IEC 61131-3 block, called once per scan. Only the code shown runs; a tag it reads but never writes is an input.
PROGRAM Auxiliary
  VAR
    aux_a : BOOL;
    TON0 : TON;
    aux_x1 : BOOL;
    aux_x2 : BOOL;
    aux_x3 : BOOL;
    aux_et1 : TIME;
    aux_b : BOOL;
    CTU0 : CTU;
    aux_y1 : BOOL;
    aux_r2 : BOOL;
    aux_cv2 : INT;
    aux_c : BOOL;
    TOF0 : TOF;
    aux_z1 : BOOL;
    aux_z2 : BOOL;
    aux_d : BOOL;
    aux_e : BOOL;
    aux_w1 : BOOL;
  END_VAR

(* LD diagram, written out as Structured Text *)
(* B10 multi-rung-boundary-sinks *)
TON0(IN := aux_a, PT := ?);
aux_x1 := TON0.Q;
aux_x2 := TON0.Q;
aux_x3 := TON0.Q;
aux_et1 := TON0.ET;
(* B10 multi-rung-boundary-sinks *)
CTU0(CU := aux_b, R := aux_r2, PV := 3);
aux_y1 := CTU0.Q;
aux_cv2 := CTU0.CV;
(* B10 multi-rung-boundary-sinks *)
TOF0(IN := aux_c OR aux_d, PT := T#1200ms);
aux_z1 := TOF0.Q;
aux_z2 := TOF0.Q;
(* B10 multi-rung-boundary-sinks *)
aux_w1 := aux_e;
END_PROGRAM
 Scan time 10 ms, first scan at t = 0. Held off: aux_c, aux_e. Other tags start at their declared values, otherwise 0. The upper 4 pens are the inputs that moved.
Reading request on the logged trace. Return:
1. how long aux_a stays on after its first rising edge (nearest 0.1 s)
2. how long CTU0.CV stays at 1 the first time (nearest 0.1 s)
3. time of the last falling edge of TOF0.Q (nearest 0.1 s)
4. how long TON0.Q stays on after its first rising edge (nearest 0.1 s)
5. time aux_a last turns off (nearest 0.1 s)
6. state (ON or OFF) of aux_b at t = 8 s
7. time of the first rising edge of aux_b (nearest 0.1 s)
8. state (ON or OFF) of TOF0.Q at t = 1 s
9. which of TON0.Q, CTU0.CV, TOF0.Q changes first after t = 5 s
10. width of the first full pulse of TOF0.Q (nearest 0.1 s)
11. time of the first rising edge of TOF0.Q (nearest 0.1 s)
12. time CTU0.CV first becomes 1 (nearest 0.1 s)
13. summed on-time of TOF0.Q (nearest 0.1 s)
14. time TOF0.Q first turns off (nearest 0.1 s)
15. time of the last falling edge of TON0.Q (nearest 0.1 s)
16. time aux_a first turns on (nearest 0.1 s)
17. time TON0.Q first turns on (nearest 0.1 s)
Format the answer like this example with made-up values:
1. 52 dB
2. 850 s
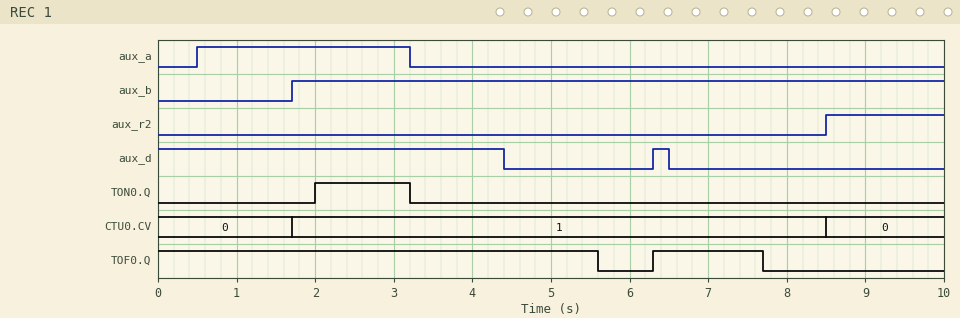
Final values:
1. 2.7 s
2. 6.8 s
3. 7.7 s
4. 1.2 s
5. 3.2 s
6. ON
7. 1.7 s
8. ON
9. TOF0.Q
10. 1.4 s
11. 6.3 s
12. 1.7 s
13. 7.0 s
14. 5.6 s
15. 3.2 s
16. 0.5 s
17. 2.0 s
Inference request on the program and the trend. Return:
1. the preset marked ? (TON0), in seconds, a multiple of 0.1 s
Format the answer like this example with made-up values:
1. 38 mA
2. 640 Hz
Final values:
1. 1.5 s
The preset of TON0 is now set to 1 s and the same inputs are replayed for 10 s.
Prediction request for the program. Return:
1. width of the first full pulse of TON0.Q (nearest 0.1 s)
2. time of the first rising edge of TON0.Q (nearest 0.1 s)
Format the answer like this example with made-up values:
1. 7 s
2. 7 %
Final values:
1. 1.7 s
2. 1.5 s
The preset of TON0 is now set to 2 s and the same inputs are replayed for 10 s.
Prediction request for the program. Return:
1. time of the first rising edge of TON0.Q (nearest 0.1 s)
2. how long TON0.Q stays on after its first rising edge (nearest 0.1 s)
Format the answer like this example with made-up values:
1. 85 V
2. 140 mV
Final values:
1. 2.5 s
2. 0.7 s
